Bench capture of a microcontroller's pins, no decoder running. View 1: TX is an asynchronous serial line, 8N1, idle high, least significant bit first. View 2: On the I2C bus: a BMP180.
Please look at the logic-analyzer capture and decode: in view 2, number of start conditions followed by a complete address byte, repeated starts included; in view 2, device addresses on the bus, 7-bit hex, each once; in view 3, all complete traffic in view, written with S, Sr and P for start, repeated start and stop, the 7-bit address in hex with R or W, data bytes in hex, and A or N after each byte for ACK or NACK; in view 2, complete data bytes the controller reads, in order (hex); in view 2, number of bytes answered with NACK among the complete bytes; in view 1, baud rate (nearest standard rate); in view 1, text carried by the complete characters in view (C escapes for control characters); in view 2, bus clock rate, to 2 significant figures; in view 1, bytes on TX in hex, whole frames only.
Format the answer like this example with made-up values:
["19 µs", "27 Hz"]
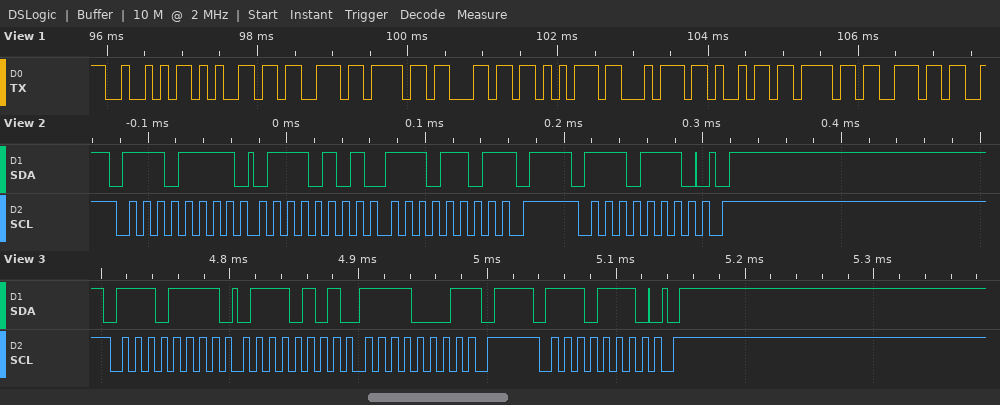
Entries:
["2", "0x77", "S 77R A 75 A F1 N P S 77W A P", "75 ED", "1", "9600 baud", "\"Resolution\"", "100 kHz", "52 65 73 6F 6C 75 74 69 6F 6E"]
